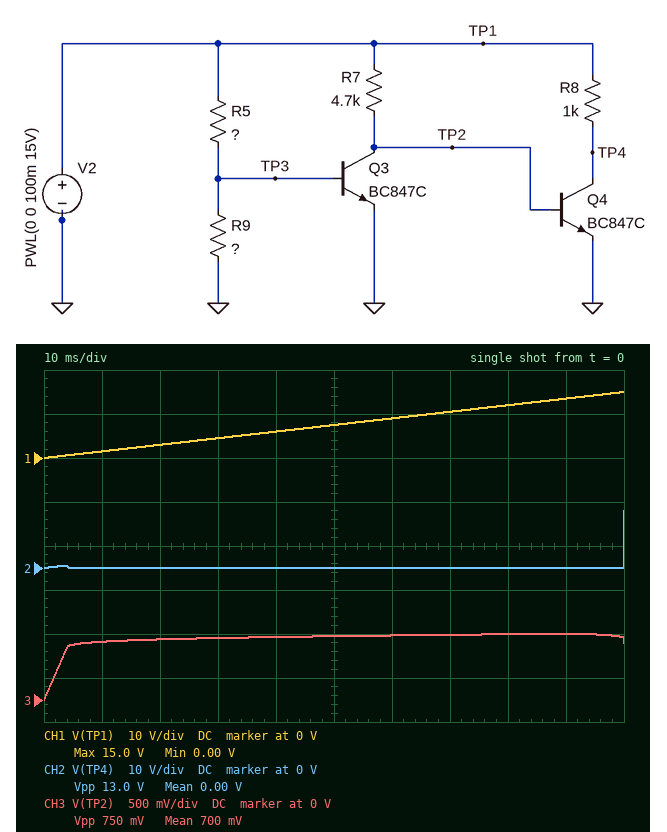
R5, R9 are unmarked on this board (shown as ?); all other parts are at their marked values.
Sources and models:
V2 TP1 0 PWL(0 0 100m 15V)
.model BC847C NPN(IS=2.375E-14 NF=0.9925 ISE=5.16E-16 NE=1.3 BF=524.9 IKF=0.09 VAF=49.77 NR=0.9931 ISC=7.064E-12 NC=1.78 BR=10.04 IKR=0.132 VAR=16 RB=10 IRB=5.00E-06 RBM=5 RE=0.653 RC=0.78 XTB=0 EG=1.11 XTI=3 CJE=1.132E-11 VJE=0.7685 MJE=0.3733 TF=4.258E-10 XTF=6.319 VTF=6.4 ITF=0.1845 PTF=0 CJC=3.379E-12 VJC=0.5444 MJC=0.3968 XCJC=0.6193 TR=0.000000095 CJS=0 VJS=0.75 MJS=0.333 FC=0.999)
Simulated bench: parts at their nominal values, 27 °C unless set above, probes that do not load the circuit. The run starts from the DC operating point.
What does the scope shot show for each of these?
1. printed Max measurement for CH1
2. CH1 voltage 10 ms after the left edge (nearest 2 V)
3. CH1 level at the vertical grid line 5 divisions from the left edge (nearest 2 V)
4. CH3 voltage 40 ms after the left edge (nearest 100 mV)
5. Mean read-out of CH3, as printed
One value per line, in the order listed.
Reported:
15.0 V
2 V
8 V
700 mV
700 mV
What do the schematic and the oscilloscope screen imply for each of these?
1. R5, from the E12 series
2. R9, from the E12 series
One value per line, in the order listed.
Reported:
3.9 kΩ
180 Ω
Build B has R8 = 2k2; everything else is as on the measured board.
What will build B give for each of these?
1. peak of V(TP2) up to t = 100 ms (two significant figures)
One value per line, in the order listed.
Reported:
740 mV
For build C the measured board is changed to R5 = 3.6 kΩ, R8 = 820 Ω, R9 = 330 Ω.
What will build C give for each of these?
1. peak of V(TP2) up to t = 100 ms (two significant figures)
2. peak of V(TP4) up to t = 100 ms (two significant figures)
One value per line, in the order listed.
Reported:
720 mV
15 V
